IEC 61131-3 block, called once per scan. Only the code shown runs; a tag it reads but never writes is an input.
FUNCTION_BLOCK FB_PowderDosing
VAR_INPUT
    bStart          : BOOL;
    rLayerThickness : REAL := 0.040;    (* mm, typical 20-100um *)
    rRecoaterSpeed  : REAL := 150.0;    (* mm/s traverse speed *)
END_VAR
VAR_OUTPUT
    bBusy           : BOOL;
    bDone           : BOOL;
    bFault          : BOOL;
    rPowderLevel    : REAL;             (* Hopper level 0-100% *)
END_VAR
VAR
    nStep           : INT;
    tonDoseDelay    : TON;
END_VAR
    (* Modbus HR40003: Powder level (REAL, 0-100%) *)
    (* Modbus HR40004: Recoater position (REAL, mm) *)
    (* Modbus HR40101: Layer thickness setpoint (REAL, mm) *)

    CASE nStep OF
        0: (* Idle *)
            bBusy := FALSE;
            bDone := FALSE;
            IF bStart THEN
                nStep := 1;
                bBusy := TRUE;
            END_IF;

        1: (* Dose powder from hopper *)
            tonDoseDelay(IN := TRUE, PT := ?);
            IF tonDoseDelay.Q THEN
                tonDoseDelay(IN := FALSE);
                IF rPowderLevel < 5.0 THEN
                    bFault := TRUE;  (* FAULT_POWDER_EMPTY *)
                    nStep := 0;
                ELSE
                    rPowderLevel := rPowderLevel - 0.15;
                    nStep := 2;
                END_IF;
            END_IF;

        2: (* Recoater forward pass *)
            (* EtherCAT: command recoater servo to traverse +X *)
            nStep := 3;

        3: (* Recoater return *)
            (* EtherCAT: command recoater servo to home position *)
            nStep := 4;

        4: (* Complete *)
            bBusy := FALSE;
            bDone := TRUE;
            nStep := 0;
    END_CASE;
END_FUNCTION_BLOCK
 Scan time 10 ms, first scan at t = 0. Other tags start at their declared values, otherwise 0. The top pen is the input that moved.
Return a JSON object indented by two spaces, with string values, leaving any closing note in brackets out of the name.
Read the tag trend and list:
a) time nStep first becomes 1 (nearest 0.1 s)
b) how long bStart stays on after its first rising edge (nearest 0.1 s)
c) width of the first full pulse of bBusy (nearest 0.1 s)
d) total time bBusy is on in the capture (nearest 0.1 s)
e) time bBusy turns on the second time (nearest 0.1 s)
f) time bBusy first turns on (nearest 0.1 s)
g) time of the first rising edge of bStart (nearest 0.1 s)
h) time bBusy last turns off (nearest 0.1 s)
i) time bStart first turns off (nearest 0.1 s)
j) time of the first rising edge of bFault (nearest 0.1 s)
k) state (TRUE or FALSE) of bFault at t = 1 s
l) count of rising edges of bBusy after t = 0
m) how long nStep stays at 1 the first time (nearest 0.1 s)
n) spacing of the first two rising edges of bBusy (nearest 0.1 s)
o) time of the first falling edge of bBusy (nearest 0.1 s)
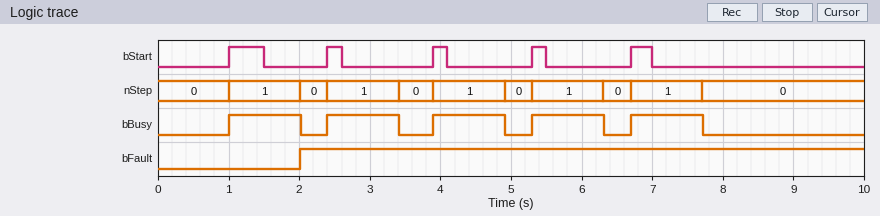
{
  "time nStep first becomes 1": "1.0 s",
  "how long bStart stays on after its first rising edge": "0.5 s",
  "width of the first full pulse of bBusy": "1.0 s",
  "total time bBusy is on in the capture": "5.1 s",
  "time bBusy turns on the second time": "2.4 s",
  "time bBusy first turns on": "1.0 s",
  "time of the first rising edge of bStart": "1.0 s",
  "time bBusy last turns off": "7.7 s",
  "time bStart first turns off": "1.5 s",
  "time of the first rising edge of bFault": "2.0 s",
  "state (TRUE or FALSE) of bFault at t = 1 s": "FALSE",
  "count of rising edges of bBusy after t = 0": "5",
  "how long nStep stays at 1 the first time": "1.0 s",
  "spacing of the first two rising edges of bBusy": "1.4 s",
  "time of the first falling edge of bBusy": "2.0 s"
}
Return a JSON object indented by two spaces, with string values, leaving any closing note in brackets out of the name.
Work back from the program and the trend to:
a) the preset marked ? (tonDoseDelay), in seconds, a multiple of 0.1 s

{
  "the preset marked ? (tonDoseDelay), in seconds, a multiple of 0.1 s": "1.0 s"
}
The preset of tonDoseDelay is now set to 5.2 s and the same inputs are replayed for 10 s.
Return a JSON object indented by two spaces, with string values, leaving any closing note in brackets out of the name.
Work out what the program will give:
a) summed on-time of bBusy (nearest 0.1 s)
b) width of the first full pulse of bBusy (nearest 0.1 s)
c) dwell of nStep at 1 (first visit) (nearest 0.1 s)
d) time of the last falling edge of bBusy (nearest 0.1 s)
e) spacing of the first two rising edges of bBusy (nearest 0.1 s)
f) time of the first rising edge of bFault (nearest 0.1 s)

{
  "summed on-time of bBusy": "8.5 s",
  "width of the first full pulse of bBusy": "5.2 s",
  "dwell of nStep at 1 (first visit)": "5.2 s",
  "time of the last falling edge of bBusy": "6.2 s",
  "spacing of the first two rising edges of bBusy": "5.7 s",
  "time of the first rising edge of bFault": "6.2 s"
}
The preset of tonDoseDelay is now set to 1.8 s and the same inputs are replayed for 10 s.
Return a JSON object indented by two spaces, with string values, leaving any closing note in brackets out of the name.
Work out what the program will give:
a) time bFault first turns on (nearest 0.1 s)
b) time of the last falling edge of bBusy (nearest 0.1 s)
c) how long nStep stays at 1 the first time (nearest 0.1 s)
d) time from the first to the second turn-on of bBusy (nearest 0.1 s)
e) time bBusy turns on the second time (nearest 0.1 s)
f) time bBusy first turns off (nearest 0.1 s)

{
  "time bFault first turns on": "2.8 s",
  "time of the last falling edge of bBusy": "8.5 s",
  "how long nStep stays at 1 the first time": "1.8 s",
  "time from the first to the second turn-on of bBusy": "2.9 s",
  "time bBusy turns on the second time": "3.9 s",
  "time bBusy first turns off": "2.8 s"
}
